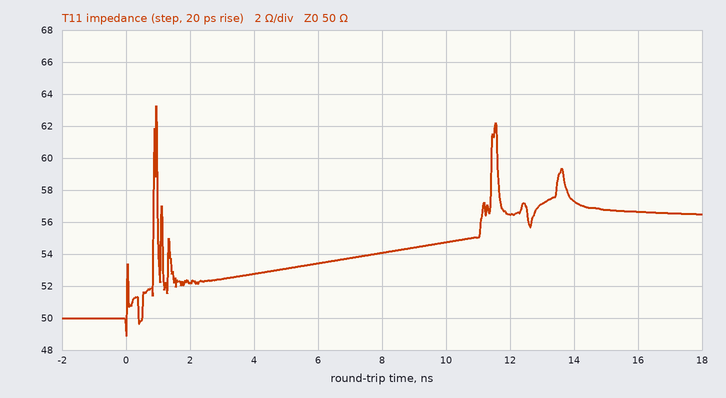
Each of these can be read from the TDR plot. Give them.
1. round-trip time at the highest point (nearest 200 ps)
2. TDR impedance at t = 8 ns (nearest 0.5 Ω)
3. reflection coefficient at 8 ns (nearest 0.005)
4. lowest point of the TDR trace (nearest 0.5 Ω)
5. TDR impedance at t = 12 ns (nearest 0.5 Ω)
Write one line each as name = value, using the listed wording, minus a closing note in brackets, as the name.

round-trip time at the highest point = 1.0 ns
TDR impedance at t = 8 ns = 54.0 Ω
reflection coefficient at 8 ns = +0.040
lowest point of the TDR trace = 49.0 Ω
TDR impedance at t = 12 ns = 56.5 Ω
